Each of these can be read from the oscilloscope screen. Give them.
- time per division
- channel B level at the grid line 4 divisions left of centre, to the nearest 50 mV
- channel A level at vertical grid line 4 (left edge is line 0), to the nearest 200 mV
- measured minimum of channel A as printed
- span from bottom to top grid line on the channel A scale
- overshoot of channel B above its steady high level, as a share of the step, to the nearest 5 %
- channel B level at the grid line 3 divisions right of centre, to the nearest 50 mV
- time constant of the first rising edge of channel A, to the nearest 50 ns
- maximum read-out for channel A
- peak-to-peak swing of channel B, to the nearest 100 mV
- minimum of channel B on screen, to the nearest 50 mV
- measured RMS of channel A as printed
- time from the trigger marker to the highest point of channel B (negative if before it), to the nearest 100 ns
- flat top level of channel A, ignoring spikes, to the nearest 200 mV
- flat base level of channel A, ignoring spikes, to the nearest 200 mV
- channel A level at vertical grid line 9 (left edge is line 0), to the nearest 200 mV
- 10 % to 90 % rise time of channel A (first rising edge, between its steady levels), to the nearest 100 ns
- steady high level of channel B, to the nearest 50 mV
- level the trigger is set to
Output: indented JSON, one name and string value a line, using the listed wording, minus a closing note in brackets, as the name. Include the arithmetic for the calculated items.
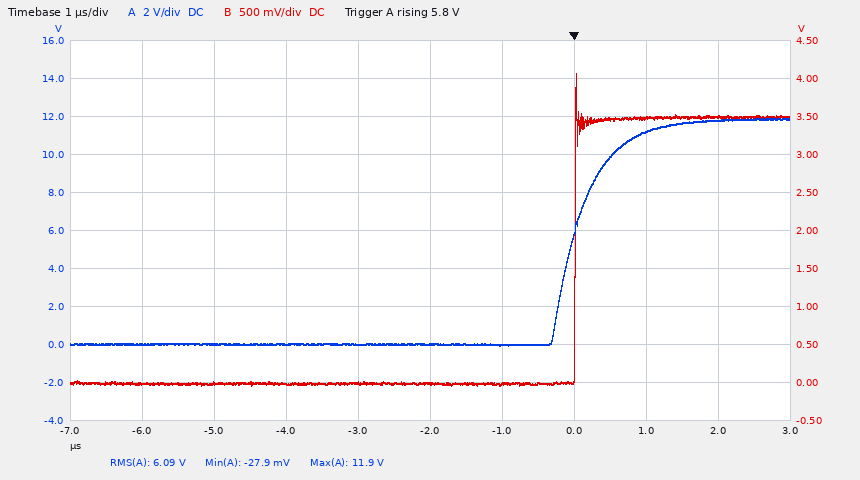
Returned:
{
  "time per division": "1 µs",
  "channel B level at the grid line 4 divisions left of centre, to the nearest 50 mV": "0 mV",
  "channel A level at vertical grid line 4 (left edge is line 0), to the nearest 200 mV": "0.0 V",
  "measured minimum of channel A as printed": "-27.9 mV",
  "span from bottom to top grid line on the channel A scale": "20 V",
  "overshoot of channel B above its steady high level, as a share of the step, to the nearest 5 %": "15 %",
  "channel B level at the grid line 3 divisions right of centre, to the nearest 50 mV": "3.50 V",
  "time constant of the first rising edge of channel A, to the nearest 50 ns": "1.0 µs / 2.2 ≈ 455 ns, so 450 ns to the nearest 50 ns",
  "maximum read-out for channel A": "11.9 V",
  "peak-to-peak swing of channel B, to the nearest 100 mV": "4.10 V",
  "minimum of channel B on screen, to the nearest 50 mV": "-50 mV",
  "measured RMS of channel A as printed": "6.09 V",
  "time from the trigger marker to the highest point of channel B (negative if before it), to the nearest 100 ns": "0.0 µs",
  "flat top level of channel A, ignoring spikes, to the nearest 200 mV": "11.8 V",
  "flat base level of channel A, ignoring spikes, to the nearest 200 mV": "0.0 V",
  "channel A level at vertical grid line 9 (left edge is line 0), to the nearest 200 mV": "11.8 V",
  "10 % to 90 % rise time of channel A (first rising edge, between its steady levels), to the nearest 100 ns": "1.0 µs",
  "steady high level of channel B, to the nearest 50 mV": "3.50 V",
  "level the trigger is set to": "5.8 V"
}
